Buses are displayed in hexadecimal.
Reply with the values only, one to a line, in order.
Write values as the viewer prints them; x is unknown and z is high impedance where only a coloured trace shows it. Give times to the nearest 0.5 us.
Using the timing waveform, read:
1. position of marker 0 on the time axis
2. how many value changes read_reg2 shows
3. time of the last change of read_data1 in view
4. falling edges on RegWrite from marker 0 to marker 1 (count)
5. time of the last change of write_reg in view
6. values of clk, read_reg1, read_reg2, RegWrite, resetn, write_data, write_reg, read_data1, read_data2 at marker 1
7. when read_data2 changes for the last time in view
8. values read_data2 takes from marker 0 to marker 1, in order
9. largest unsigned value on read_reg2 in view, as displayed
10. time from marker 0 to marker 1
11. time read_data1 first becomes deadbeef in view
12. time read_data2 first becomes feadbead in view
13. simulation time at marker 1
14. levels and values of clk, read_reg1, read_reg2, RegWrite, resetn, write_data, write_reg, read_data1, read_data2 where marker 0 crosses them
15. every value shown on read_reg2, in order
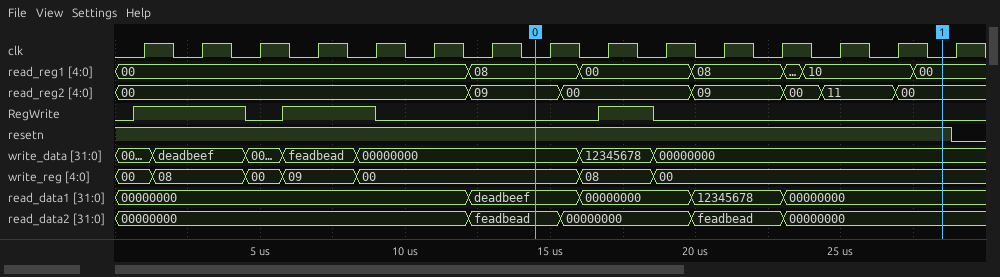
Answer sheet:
14.5 us
6
23 us
1
18.5 us
clk=0, read_reg1=00, read_reg2=00, RegWrite=0, resetn=1, write_data=00000000, write_reg=00, read_data1=00000000, read_data2=00000000
23 us
feadbead, 00000000, feadbead, 00000000
11
14 us
12 us
12 us
28.5 us
clk=0, read_reg1=08, read_reg2=09, RegWrite=0, resetn=1, write_data=00000000, write_reg=00, read_data1=deadbeef, read_data2=feadbead
00, 09, 00, 09, 00, 11, 00
